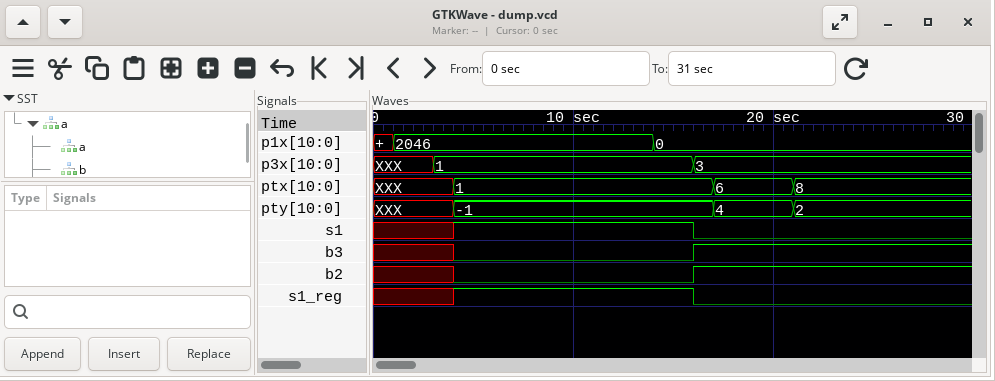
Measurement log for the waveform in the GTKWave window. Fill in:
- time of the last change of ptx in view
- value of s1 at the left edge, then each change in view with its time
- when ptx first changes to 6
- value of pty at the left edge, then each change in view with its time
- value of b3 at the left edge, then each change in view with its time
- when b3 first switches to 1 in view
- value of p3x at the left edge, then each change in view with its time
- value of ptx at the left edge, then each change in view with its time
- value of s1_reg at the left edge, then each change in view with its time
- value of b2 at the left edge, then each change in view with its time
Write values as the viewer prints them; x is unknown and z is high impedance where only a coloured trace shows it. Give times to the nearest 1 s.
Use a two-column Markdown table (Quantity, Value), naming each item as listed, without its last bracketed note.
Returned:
| Quantity | Value |
|---|---|
| time of the last change of ptx in view | 21 s |
| value of s1 at the left edge, then each change in view with its time | x, 1 at 4 s, 0 at 16 s |
| when ptx first changes to 6 | 17 s |
| value of pty at the left edge, then each change in view with its time | XXX, -1 at 4 s, 4 at 17 s, 2 at 21 s |
| value of b3 at the left edge, then each change in view with its time | x, 0 at 4 s, 1 at 16 s |
| when b3 first switches to 1 in view | 16 s |
| value of p3x at the left edge, then each change in view with its time | XXX, 1 at 3 s, 3 at 16 s |
| value of ptx at the left edge, then each change in view with its time | XXX, 1 at 4 s, 6 at 17 s, 8 at 21 s |
| value of s1_reg at the left edge, then each change in view with its time | x, 1 at 4 s, 0 at 16 s |
| value of b2 at the left edge, then each change in view with its time | x, 0 at 4 s, 1 at 16 s |
